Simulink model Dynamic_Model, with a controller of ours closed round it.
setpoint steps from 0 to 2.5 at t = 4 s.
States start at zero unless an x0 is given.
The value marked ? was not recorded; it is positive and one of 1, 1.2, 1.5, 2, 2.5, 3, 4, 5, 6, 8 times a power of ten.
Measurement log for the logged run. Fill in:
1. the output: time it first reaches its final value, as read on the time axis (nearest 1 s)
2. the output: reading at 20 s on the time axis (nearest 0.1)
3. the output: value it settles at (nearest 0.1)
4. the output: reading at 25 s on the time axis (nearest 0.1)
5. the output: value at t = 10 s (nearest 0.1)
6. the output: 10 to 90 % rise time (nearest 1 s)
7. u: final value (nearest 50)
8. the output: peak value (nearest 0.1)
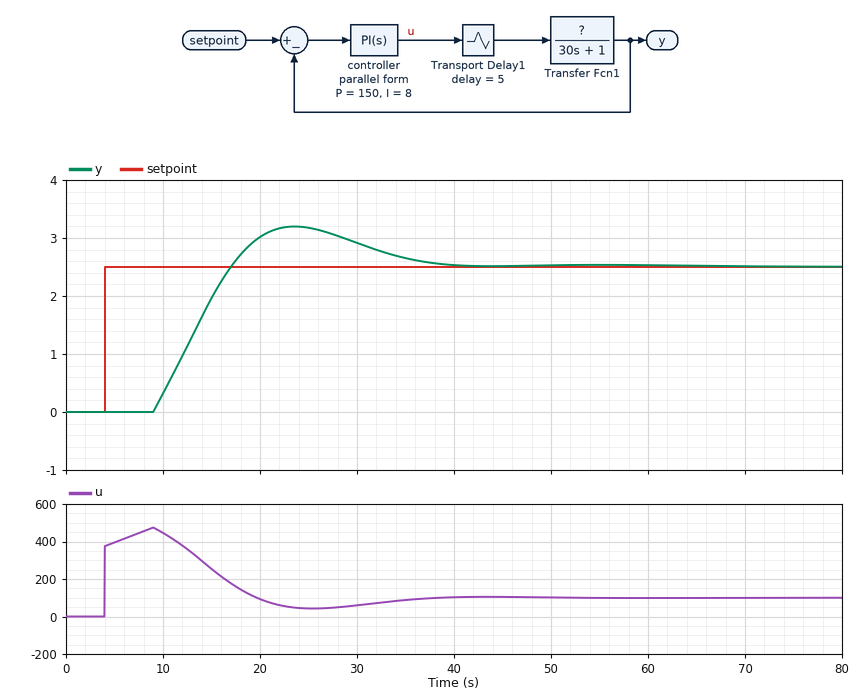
17 s
3.0
2.5
3.2
0.3
6 s
100
3.2
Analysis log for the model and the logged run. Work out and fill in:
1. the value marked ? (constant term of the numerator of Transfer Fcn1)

0.025
